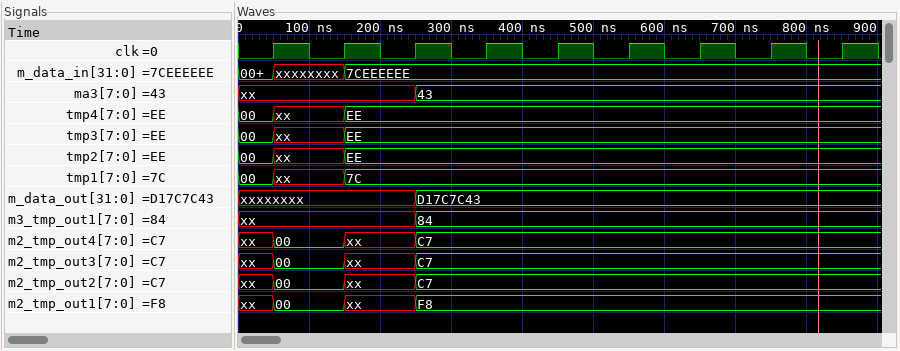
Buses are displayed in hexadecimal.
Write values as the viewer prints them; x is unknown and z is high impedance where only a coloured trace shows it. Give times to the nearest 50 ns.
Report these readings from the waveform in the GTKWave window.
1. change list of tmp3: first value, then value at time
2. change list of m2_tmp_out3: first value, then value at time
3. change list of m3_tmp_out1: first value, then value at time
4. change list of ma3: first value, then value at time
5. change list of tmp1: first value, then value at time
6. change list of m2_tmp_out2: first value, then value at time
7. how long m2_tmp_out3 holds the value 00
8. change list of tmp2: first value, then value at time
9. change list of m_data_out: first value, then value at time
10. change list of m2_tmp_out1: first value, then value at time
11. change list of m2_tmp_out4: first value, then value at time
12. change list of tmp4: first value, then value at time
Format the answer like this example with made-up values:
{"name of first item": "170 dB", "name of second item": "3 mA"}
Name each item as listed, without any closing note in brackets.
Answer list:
{"change list of tmp3: first value, then value at time": "00, xx at 50 ns, EE at 150 ns", "change list of m2_tmp_out3: first value, then value at time": "xx, 00 at 50 ns, xx at 150 ns, C7 at 250 ns", "change list of m3_tmp_out1: first value, then value at time": "xx, 84 at 250 ns", "change list of ma3: first value, then value at time": "xx, 43 at 250 ns", "change list of tmp1: first value, then value at time": "00, xx at 50 ns, 7C at 150 ns", "change list of m2_tmp_out2: first value, then value at time": "xx, 00 at 50 ns, xx at 150 ns, C7 at 250 ns", "how long m2_tmp_out3 holds the value 00": "100 ns", "change list of tmp2: first value, then value at time": "00, xx at 50 ns, EE at 150 ns", "change list of m_data_out: first value, then value at time": "xxxxxxxx, D17C7C43 at 250 ns", "change list of m2_tmp_out1: first value, then value at time": "xx, 00 at 50 ns, xx at 150 ns, F8 at 250 ns", "change list of m2_tmp_out4: first value, then value at time": "xx, 00 at 50 ns, xx at 150 ns, C7 at 250 ns", "change list of tmp4: first value, then value at time": "00, xx at 50 ns, EE at 150 ns"}
